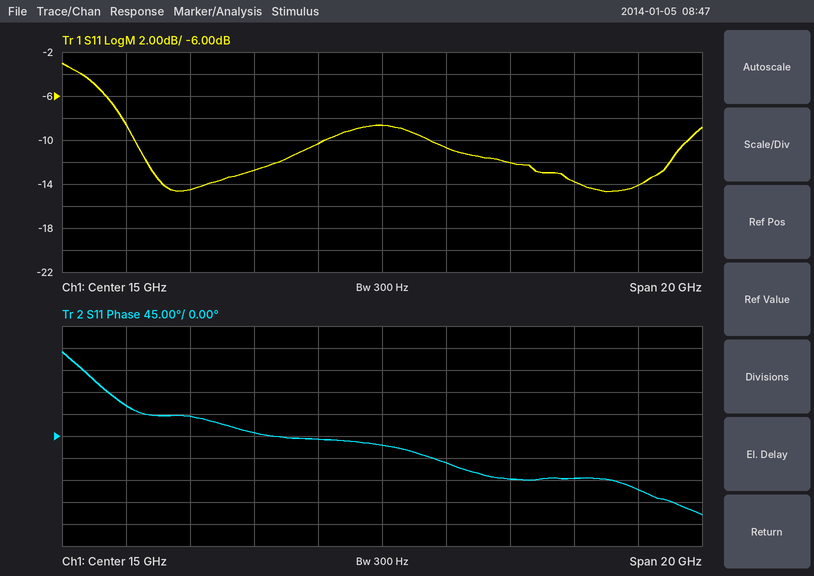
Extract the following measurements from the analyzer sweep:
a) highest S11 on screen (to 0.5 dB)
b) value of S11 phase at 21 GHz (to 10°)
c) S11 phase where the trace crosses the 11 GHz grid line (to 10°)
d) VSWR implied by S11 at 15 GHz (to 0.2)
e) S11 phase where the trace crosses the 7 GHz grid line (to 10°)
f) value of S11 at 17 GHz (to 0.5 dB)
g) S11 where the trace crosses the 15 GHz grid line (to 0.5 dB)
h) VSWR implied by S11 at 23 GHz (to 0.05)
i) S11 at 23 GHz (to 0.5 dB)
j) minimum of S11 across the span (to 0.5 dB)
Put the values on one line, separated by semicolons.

-3.0 dB; -90°; 10°; 2.2; 60°; -10.5 dB; -8.5 dB; 1.50; -14.0 dB; -14.5 dB
